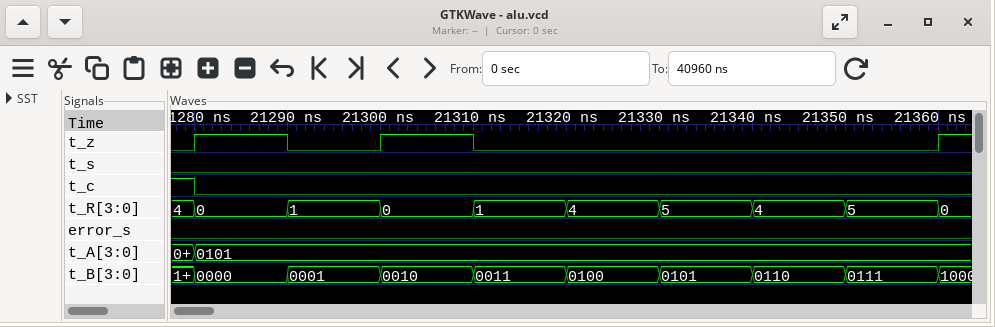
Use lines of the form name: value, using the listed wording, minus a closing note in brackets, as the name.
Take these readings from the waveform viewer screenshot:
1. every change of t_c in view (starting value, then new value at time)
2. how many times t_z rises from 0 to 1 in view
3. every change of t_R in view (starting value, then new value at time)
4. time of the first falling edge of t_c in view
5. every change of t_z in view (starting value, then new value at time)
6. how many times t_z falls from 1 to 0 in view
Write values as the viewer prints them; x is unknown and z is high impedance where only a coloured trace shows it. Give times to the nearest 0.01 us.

every change of t_c in view: 1, 0 at 21.28 us
how many times t_z rises from 0 to 1 in view: 3
every change of t_R in view: 4, 0 at 21.28 us, 1 at 21.29 us, 0 at 21.3 us, 1 at 21.31 us, 4 at 21.32 us, 5 at 21.33 us, 4 at 21.34 us, 5 at 21.35 us, 0 at 21.36 us
time of the first falling edge of t_c in view: 21.28 us
every change of t_z in view: 0, 1 at 21.28 us, 0 at 21.29 us, 1 at 21.3 us, 0 at 21.31 us, 1 at 21.36 us
how many times t_z falls from 1 to 0 in view: 2
